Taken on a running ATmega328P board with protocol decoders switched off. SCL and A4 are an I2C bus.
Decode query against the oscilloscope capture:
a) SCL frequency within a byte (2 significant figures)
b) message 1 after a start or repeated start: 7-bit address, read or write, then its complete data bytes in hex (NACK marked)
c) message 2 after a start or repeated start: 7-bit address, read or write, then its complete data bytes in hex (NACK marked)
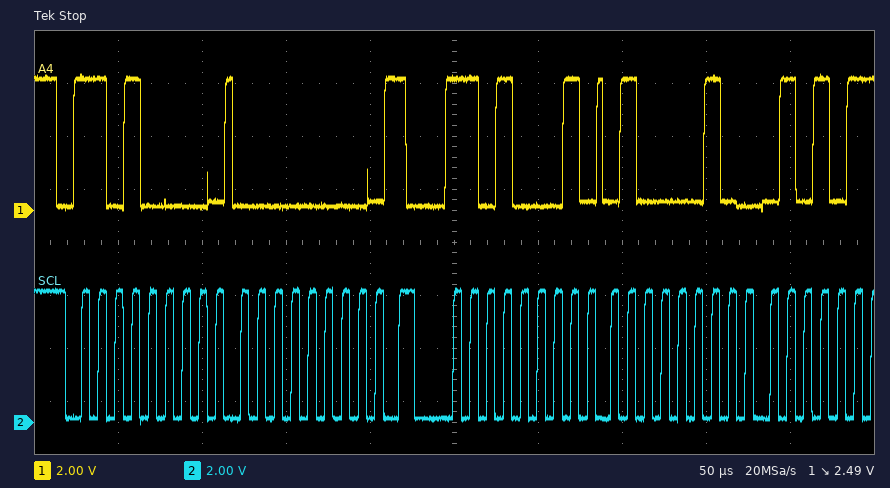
100 kHz
0x68 write: 00
0x68 read: 42
